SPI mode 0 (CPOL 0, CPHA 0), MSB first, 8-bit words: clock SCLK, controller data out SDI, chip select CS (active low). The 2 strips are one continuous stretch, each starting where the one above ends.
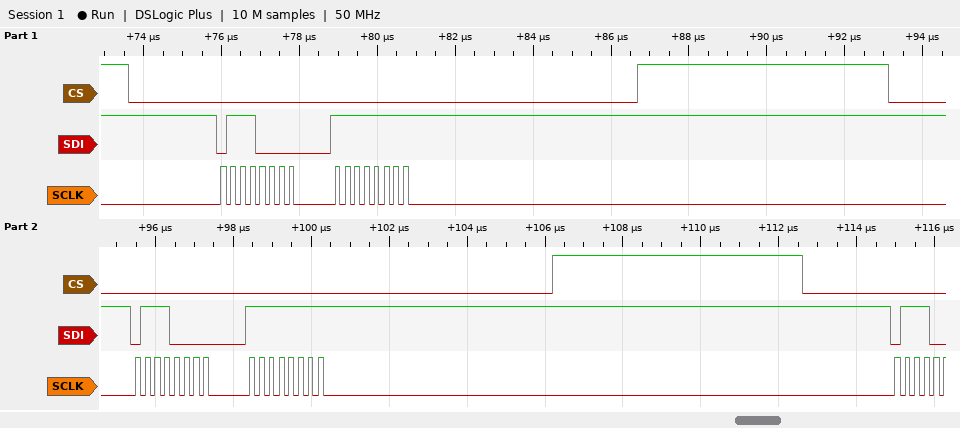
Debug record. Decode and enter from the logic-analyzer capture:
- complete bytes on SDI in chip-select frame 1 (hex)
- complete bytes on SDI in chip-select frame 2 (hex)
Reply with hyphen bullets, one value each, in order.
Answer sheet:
- 0x70 0xFF
- 0x70 0xFF
